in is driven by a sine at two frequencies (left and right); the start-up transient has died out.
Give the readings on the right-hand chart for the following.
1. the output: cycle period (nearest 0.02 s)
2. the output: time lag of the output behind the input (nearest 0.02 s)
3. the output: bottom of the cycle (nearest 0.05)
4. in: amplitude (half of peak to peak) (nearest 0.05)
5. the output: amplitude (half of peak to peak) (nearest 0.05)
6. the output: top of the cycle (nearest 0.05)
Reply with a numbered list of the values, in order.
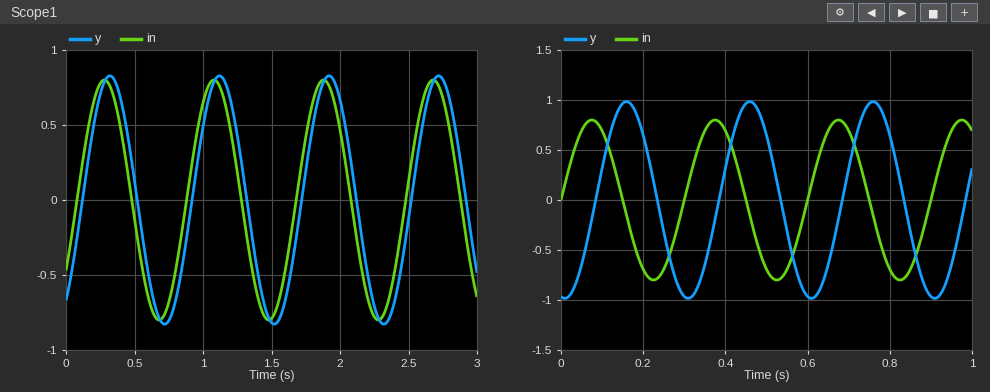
1. 0.30 s
2. 0.08 s
3. -1.00
4. 0.80
5. 1.00
6. 1.00
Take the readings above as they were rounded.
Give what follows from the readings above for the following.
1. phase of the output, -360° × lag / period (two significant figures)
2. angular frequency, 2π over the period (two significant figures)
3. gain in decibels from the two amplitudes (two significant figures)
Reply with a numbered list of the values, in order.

1. -96°
2. 21 rad/s
3. 1.9 dB
